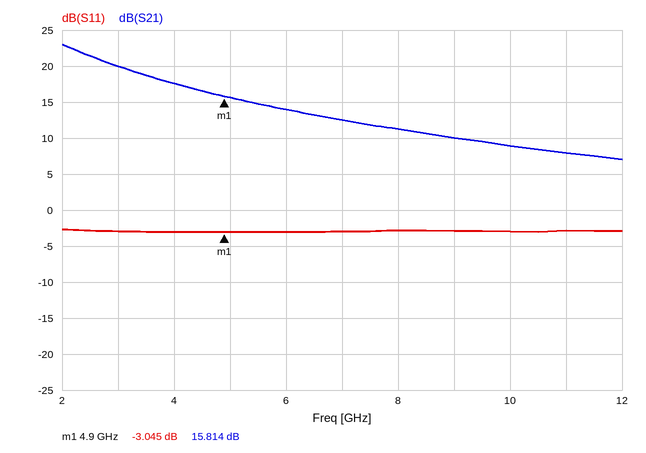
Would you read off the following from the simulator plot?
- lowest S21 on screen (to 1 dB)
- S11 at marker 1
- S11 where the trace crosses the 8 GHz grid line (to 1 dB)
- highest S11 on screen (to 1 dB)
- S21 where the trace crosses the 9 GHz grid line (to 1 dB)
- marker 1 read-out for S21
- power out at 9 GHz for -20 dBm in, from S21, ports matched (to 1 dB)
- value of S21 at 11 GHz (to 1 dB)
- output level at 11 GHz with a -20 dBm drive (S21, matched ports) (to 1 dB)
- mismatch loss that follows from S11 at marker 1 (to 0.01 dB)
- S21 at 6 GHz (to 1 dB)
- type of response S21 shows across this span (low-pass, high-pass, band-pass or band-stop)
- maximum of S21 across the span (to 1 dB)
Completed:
7 dB
-3.045 dB
-3 dB
-3 dB
10 dB
15.814 dB
-10 dBm
8 dB
-12 dBm
2.98 dB
14 dB
low-pass
23 dB
